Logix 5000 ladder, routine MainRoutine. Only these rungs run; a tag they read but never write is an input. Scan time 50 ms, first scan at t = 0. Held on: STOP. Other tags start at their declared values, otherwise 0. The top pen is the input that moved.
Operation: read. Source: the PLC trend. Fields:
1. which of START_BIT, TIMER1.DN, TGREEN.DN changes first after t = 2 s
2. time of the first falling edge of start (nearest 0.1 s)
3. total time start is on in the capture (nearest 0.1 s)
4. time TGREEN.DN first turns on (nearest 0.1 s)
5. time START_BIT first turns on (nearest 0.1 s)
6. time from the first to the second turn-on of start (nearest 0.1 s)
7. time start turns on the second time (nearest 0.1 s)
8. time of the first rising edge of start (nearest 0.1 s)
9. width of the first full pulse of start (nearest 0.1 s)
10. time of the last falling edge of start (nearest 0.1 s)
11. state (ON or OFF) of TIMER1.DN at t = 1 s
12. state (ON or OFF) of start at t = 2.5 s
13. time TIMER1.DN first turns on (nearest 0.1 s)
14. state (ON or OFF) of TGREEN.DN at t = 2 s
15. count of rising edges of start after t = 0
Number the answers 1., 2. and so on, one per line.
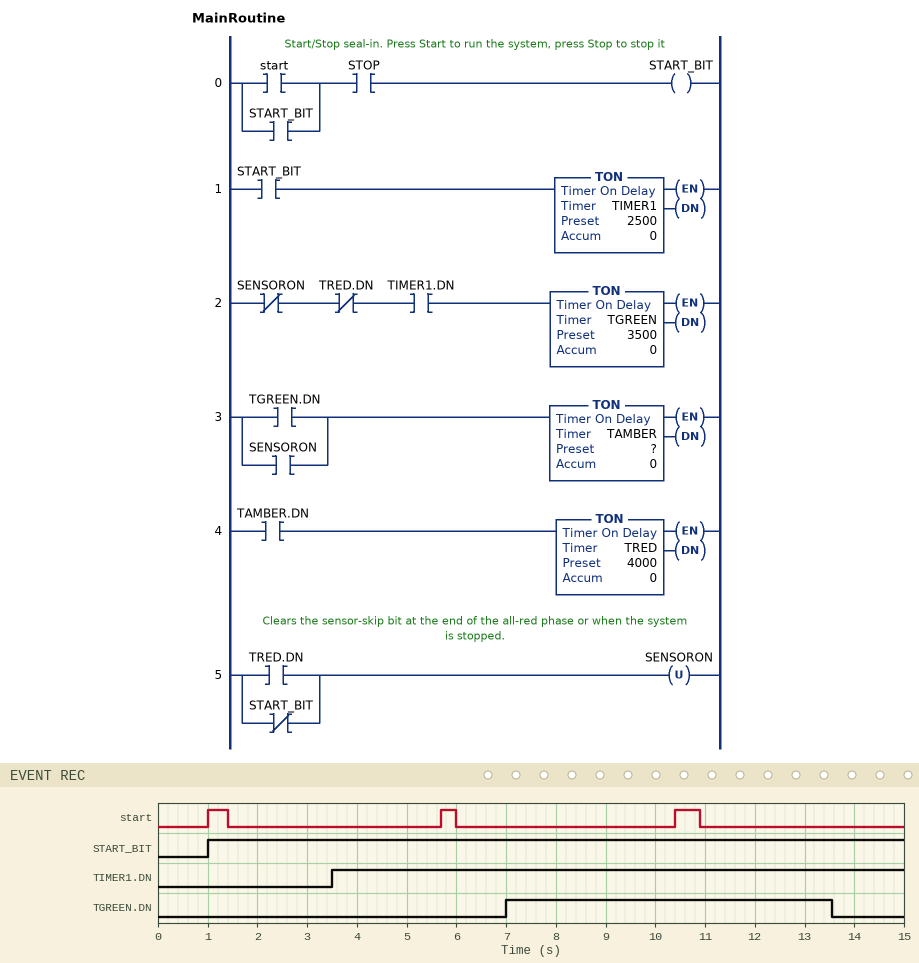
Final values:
1. TIMER1.DN
2. 1.4 s
3. 1.2 s
4. 7.0 s
5. 1.0 s
6. 4.7 s
7. 5.7 s
8. 1.0 s
9. 0.4 s
10. 10.9 s
11. OFF
12. OFF
13. 3.5 s
14. OFF
15. 3
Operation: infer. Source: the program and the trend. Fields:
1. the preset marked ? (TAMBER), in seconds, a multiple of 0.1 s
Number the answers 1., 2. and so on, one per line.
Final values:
1. 2.5 s
